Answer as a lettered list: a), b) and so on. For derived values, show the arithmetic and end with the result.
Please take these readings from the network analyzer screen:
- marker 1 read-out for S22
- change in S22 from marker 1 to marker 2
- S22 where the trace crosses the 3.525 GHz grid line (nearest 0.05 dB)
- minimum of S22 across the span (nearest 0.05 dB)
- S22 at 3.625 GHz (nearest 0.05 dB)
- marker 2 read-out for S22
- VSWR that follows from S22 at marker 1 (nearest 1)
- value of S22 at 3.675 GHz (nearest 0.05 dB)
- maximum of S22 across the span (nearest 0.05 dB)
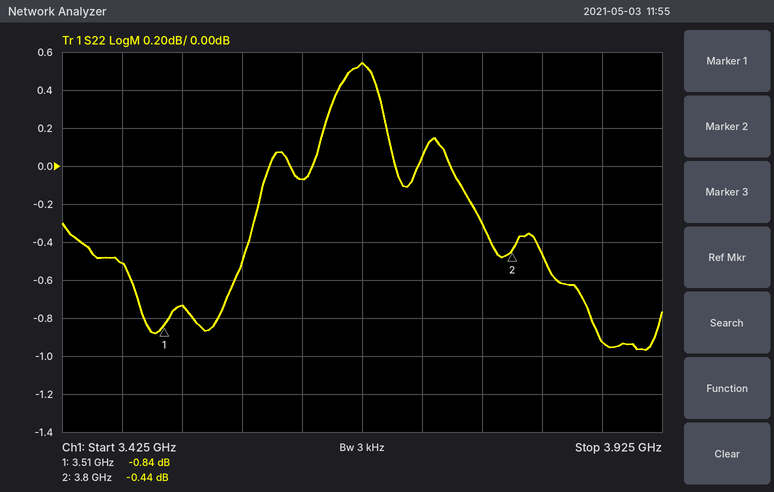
a) -0.84 dB
b) -0.44 − (-0.84) = 0.40 dB
c) -0.75 dB
d) -0.95 dB
e) -0.05 dB
f) -0.44 dB
g) (1 + 0.9078)/(1 − 0.9078) ≈ 21
h) 0.55 dB
i) 0.55 dB
